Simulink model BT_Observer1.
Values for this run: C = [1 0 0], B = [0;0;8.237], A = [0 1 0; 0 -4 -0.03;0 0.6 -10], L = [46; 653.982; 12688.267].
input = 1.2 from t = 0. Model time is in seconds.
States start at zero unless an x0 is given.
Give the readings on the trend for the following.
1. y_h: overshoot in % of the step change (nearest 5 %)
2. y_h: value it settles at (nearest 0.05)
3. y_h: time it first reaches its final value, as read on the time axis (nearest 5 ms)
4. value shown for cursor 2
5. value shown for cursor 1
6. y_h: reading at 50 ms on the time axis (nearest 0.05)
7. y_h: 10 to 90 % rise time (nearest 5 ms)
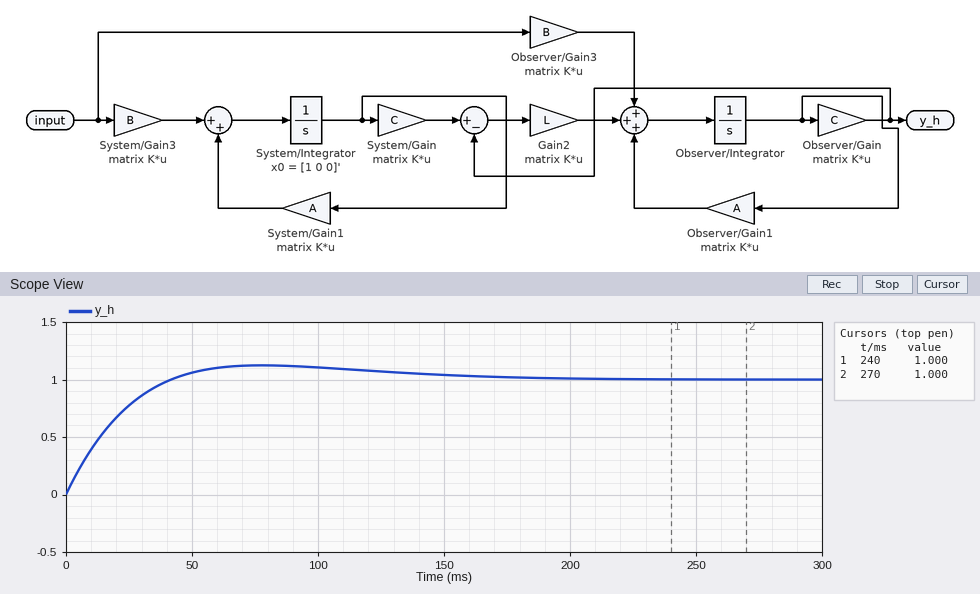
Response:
15 %
1.00
40 ms
1.000
1.000
1.05
30 ms
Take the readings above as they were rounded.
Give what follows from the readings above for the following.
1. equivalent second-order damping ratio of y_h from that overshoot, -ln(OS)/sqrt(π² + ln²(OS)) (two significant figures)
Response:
0.52
